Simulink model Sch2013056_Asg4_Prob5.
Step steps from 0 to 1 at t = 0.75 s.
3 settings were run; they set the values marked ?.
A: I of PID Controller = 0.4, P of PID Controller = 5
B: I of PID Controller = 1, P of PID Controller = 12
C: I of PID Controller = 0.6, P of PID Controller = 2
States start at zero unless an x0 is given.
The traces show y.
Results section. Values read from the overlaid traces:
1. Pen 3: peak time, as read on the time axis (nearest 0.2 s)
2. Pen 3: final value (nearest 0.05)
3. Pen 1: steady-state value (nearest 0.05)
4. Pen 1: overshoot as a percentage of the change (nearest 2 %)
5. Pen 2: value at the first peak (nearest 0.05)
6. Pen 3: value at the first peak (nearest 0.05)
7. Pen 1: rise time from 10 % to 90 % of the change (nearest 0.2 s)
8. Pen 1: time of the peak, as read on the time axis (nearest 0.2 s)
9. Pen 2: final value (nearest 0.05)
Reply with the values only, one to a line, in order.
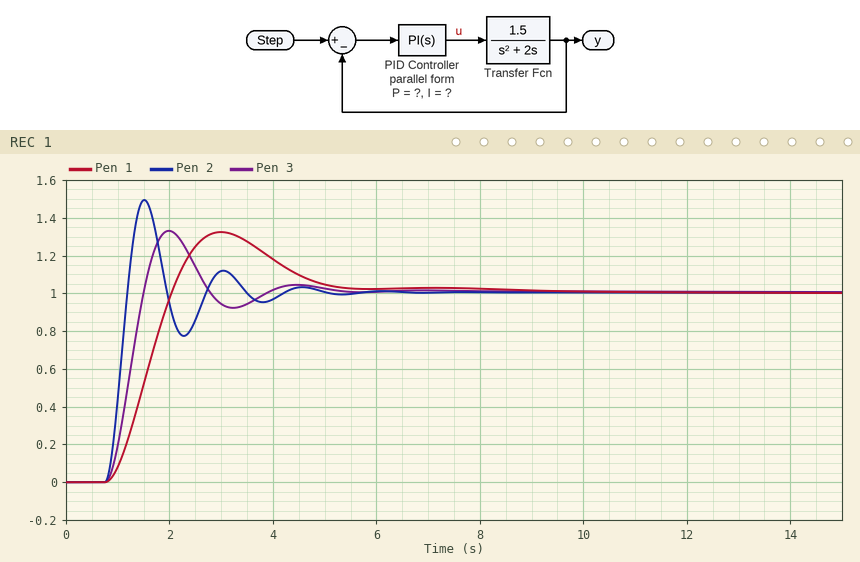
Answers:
2.0 s
1.00
1.00
32 %
1.50
1.35
0.8 s
3.0 s
1.00
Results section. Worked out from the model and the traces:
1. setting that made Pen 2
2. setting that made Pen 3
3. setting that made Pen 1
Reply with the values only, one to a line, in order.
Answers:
B
A
C
